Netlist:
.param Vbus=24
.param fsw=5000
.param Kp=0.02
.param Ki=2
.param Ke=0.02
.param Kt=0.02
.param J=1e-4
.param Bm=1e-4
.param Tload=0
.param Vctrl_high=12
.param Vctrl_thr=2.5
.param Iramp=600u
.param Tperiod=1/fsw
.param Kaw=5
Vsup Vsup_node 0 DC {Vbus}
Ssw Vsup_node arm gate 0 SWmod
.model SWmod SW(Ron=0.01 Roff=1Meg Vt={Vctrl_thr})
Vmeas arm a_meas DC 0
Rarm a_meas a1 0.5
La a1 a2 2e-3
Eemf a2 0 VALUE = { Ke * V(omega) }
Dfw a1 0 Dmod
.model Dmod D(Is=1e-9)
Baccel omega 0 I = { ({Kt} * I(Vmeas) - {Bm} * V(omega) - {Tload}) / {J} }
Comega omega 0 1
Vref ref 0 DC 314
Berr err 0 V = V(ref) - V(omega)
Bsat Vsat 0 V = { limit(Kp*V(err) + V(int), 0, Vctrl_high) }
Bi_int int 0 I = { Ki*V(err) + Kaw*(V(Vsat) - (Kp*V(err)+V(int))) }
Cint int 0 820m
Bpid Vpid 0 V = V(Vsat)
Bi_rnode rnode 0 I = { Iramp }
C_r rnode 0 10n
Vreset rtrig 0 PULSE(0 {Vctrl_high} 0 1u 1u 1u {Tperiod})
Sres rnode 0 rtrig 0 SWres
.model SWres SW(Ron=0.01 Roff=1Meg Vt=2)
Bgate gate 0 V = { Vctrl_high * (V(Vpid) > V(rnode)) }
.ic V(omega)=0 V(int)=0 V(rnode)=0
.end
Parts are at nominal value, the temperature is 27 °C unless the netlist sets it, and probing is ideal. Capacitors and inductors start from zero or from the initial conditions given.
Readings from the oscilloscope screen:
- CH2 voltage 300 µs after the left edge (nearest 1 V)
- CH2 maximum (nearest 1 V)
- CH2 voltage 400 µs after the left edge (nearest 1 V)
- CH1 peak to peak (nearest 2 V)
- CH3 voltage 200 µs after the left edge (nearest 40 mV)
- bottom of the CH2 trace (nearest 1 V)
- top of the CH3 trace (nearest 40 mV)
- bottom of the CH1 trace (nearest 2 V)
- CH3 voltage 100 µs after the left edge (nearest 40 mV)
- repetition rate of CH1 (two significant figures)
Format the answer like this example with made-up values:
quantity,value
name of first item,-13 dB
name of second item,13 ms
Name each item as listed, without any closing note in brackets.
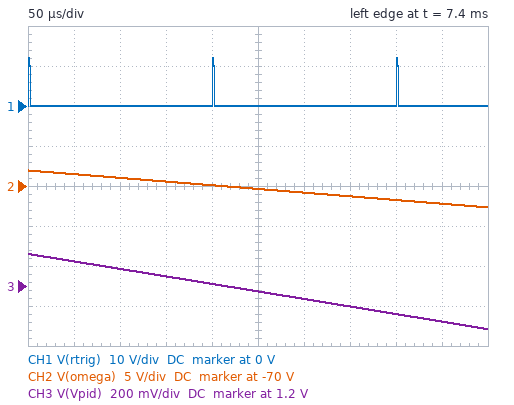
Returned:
quantity,value
CH2 voltage 300 µs after the left edge,-71 V
CH2 maximum,-68 V
CH2 voltage 400 µs after the left edge,-72 V
CH1 peak to peak,12 V
CH3 voltage 200 µs after the left edge,1.20 V
bottom of the CH2 trace,-73 V
top of the CH3 trace,1.36 V
bottom of the CH1 trace,0 V
CH3 voltage 100 µs after the left edge,1.28 V
repetition rate of CH1,5.0 kHz
